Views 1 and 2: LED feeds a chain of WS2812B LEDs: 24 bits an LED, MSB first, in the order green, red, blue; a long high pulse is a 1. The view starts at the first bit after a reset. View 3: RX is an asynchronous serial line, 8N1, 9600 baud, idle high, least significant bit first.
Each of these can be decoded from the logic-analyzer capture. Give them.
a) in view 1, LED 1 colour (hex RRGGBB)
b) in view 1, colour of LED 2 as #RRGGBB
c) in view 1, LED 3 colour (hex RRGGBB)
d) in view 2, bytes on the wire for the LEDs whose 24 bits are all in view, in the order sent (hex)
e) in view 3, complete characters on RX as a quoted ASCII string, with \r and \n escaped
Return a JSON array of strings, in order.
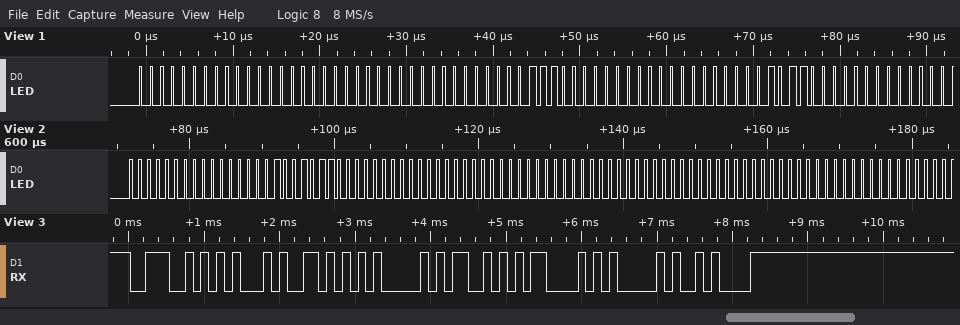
["#000000", "#0E0000", "#2C0000", "00 00 96 00 00 00 00 00 00", "\"NEVASCA\\n\""]
